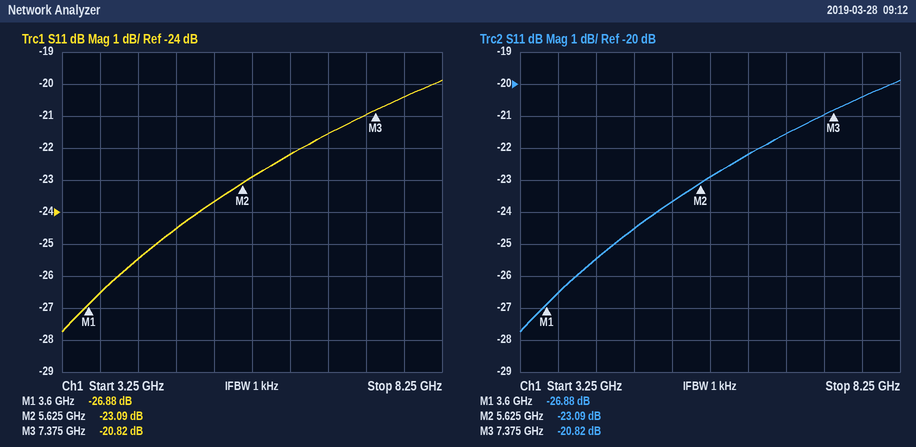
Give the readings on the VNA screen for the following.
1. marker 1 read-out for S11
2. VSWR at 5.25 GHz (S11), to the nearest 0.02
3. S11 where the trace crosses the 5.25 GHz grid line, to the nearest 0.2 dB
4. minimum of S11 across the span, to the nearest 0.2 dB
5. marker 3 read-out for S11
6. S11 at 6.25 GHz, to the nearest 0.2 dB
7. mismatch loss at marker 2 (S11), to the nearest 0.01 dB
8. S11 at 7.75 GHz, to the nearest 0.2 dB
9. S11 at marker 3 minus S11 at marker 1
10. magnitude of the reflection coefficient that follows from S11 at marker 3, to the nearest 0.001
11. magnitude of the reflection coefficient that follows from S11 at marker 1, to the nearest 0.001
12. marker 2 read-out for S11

-26.88 dB
1.14
-23.6 dB
-27.8 dB
-20.82 dB
-22.2 dB
0.02 dB
-20.4 dB
6.06 dB
0.091
0.045
-23.09 dB
